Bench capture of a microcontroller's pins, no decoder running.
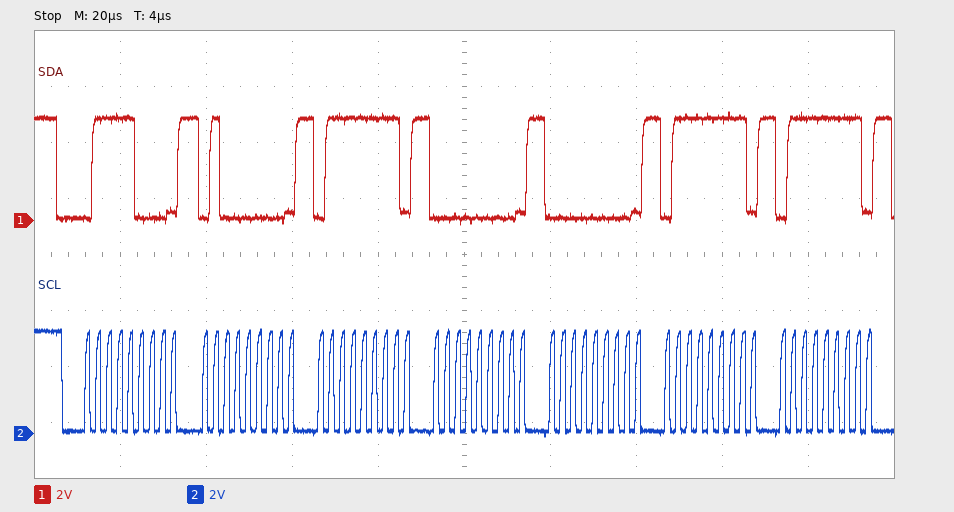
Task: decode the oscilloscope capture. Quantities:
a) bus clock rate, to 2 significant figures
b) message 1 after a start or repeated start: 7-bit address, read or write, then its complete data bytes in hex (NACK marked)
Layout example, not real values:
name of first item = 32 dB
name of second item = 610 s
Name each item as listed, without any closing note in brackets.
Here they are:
bus clock rate, to 2 significant figures = 400 kHz
message 1 after a start or repeated start: 7-bit address, read or write, then its complete data bytes in hex = 0x3C write: 40 7F 00 00 7F 7F
